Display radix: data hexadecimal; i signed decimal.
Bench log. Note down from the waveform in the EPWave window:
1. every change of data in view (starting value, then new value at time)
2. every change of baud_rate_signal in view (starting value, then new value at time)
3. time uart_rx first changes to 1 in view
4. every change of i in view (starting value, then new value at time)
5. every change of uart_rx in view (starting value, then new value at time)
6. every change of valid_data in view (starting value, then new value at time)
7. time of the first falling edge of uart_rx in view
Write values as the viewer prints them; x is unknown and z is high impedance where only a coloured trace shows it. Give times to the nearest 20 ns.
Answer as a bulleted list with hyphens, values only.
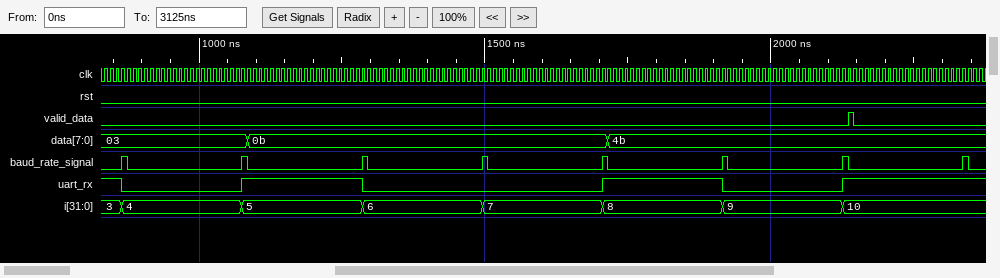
- 03, 0b at 1080 ns, 4b at 1720 ns
- 0, 1 at 860 ns, 0 at 880 ns, 1 at 1080 ns, 0 at 1080 ns, 1 at 1280 ns, 0 at 1300 ns, 1 at 1500 ns, 0 at 1500 ns, 1 at 1700 ns, 0 at 1720 ns, 1 at 1920 ns, 0 at 1920 ns, 1 at 2120 ns, 0 at 2140 ns, 1 at 2340 ns, 0 at 2340 ns
- 1080 ns
- 3, 4 at 860 ns, 5 at 1080 ns, 6 at 1280 ns, 7 at 1500 ns, 8 at 1700 ns, 9 at 1920 ns, 10 at 2120 ns
- 1, 0 at 860 ns, 1 at 1080 ns, 0 at 1280 ns, 1 at 1700 ns, 0 at 1920 ns, 1 at 2120 ns
- 0, 1 at 2140 ns, 0 at 2140 ns
- 860 ns
